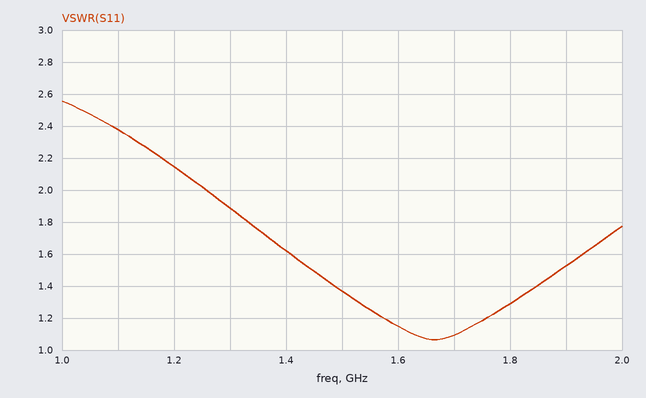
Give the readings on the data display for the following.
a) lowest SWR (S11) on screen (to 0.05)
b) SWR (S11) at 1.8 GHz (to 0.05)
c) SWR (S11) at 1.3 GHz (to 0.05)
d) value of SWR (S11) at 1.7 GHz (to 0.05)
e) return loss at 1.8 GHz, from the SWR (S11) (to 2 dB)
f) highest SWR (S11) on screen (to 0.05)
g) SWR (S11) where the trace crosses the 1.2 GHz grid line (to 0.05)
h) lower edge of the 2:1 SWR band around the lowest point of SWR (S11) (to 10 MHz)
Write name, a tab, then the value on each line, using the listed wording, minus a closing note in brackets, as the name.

lowest SWR (S11) on screen	1.05
SWR (S11) at 1.8 GHz	1.30
SWR (S11) at 1.3 GHz	1.90
value of SWR (S11) at 1.7 GHz	1.10
return loss at 1.8 GHz, from the SWR (S11)	18 dB
highest SWR (S11) on screen	2.55
SWR (S11) where the trace crosses the 1.2 GHz grid line	2.15
lower edge of the 2:1 SWR band around the lowest point of SWR (S11)	1.26 GHz
